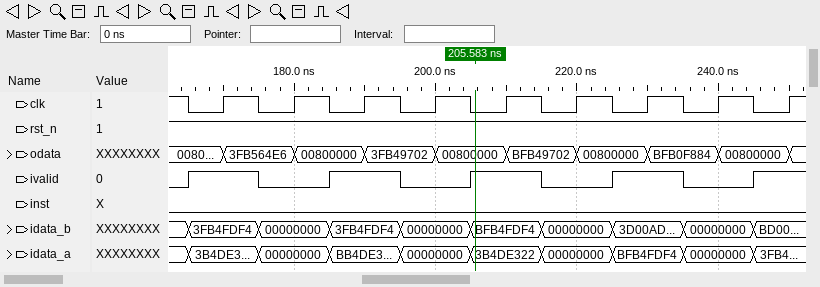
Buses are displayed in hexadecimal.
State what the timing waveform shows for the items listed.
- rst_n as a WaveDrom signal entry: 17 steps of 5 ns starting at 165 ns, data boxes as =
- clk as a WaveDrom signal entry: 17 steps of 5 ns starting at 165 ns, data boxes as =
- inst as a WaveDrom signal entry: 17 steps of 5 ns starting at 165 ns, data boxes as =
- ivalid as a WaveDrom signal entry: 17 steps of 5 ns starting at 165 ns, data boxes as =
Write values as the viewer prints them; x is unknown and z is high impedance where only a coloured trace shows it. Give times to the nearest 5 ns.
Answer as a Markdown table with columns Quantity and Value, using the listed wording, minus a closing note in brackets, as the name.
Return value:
| Quantity | Value |
|---|---|
| rst_n as a WaveDrom signal entry: 17 steps of 5 ns starting at 165 ns, data boxes as = | {name: 'rst_n', wave: '1................'} |
| clk as a WaveDrom signal entry: 17 steps of 5 ns starting at 165 ns, data boxes as = | {name: 'clk', wave: '01010101010101010'} |
| inst as a WaveDrom signal entry: 17 steps of 5 ns starting at 165 ns, data boxes as = | {name: 'inst', wave: '0................'} |
| ivalid as a WaveDrom signal entry: 17 steps of 5 ns starting at 165 ns, data boxes as = | {name: 'ivalid', wave: '1.0.1.0.1.0.1.0.1'} |
